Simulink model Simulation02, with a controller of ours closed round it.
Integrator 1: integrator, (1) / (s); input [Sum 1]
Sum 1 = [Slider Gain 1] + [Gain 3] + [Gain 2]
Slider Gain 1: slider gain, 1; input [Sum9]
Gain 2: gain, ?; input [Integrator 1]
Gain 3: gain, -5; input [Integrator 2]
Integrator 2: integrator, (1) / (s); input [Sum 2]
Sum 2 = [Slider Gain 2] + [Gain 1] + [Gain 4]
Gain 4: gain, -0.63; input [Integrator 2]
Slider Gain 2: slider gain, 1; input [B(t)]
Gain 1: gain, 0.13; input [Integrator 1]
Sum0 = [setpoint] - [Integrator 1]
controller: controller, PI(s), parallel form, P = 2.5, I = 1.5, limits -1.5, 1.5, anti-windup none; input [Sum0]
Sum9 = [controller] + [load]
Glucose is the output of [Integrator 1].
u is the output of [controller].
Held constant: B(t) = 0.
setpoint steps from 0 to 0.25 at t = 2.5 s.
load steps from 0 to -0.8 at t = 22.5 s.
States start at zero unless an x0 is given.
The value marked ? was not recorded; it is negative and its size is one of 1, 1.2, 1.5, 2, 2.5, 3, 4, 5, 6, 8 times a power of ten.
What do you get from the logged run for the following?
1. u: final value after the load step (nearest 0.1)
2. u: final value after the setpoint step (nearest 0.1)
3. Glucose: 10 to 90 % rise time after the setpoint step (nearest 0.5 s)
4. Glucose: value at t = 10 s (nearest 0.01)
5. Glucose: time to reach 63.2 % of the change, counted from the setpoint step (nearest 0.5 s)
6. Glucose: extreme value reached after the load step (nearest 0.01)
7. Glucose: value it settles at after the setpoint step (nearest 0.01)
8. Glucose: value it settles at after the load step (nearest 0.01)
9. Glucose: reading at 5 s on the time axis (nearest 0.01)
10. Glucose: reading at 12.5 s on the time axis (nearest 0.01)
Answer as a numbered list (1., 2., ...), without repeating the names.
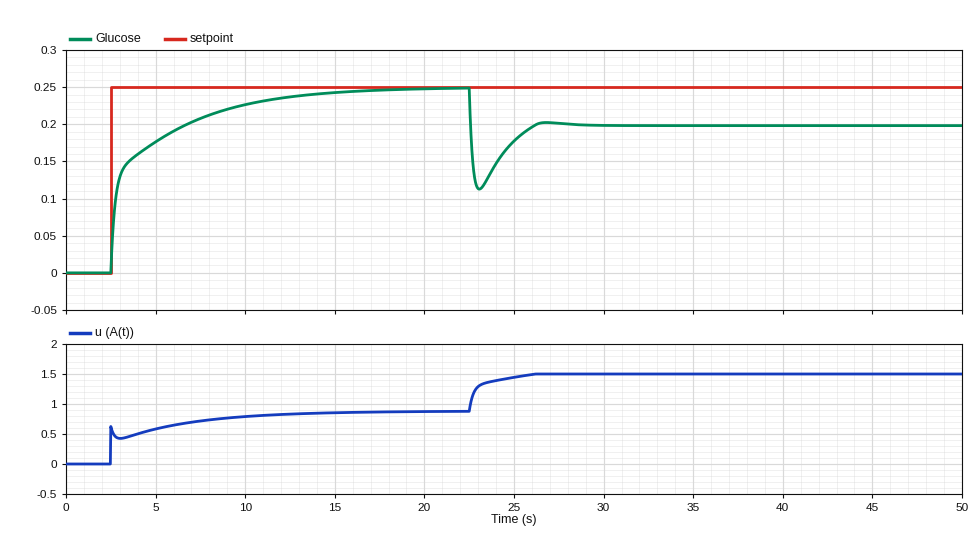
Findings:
1. 1.5
2. 0.9
3. 7.0 s
4. 0.23
5. 1.5 s
6. 0.11
7. 0.25
8. 0.20
9. 0.18
10. 0.24
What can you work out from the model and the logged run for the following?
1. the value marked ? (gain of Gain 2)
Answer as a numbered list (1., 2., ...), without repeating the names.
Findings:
1. -2.5
